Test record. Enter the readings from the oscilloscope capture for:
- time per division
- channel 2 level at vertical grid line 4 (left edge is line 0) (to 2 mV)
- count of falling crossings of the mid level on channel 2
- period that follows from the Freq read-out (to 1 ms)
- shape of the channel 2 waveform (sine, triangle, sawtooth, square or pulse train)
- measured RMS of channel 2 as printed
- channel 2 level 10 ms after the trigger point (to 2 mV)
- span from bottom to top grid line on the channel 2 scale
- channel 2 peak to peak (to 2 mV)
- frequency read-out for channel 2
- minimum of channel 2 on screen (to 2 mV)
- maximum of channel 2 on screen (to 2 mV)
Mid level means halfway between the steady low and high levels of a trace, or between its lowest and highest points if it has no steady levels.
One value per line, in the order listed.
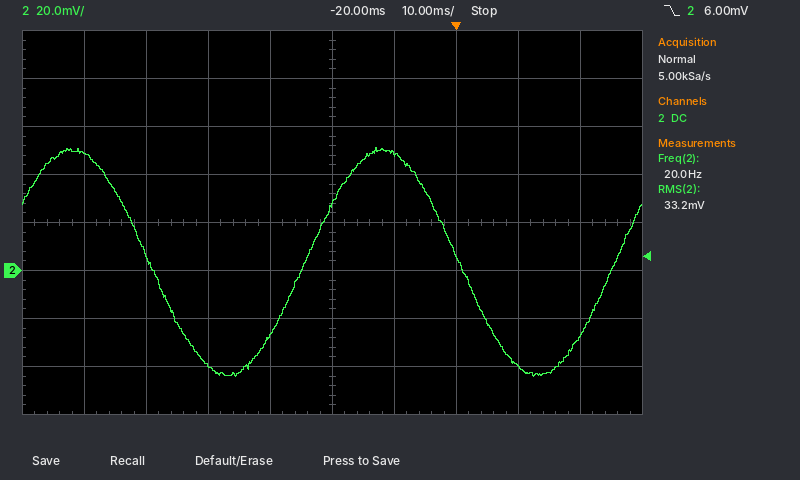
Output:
10 ms
-26 mV
2
50 ms
sine
33.2 mV
-40 mV
160 mV
96 mV
20.0 Hz
-44 mV
52 mV
